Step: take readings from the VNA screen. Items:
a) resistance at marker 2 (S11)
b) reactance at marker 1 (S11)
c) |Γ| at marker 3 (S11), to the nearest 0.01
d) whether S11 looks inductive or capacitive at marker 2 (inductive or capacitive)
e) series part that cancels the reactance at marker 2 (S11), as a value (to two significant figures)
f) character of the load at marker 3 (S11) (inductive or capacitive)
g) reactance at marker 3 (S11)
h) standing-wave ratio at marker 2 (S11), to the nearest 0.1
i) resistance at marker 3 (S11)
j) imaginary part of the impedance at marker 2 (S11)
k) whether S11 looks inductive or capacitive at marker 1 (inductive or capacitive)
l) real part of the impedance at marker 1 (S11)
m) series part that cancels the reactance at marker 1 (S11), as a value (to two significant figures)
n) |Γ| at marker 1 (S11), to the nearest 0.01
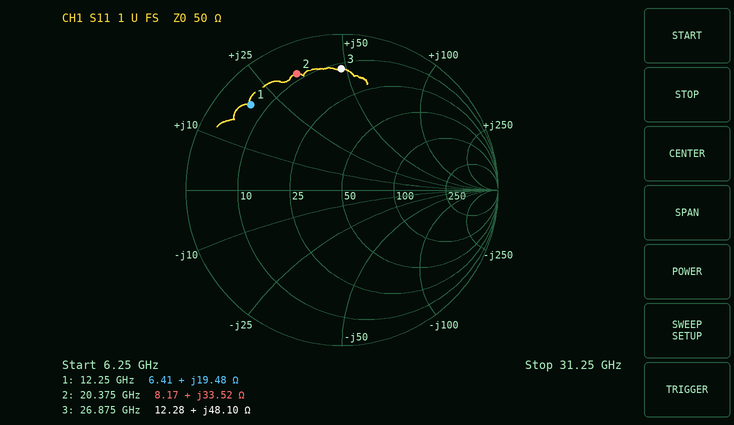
8.17 Ω
+19.48 Ω
0.78
inductive
230 fF
inductive
+48.10 Ω
8.9
12.28 Ω
+33.52 Ω
inductive
6.41 Ω
670 fF
0.80
